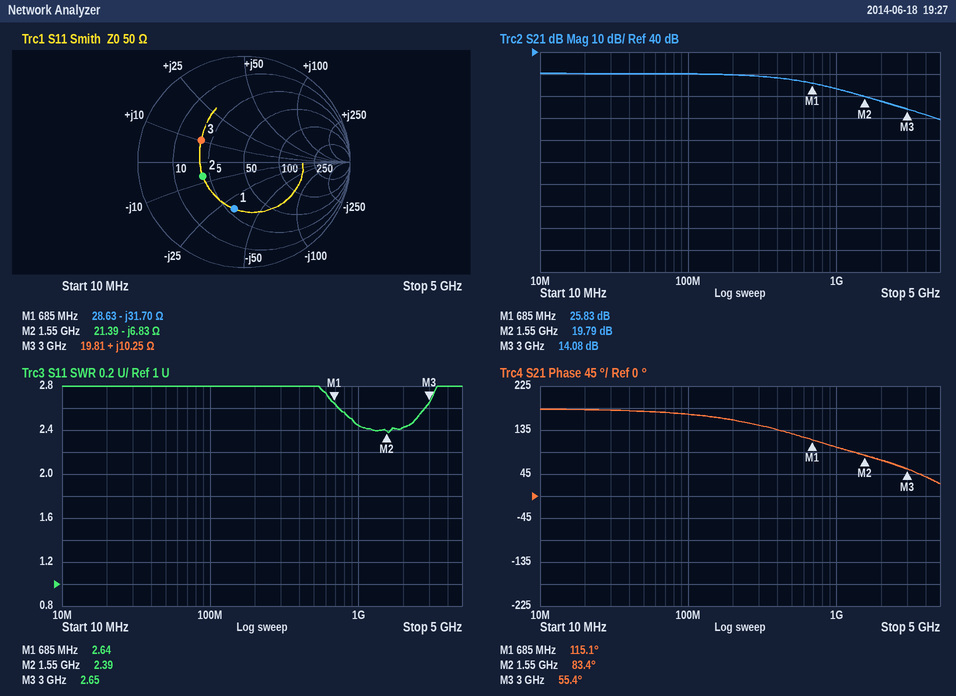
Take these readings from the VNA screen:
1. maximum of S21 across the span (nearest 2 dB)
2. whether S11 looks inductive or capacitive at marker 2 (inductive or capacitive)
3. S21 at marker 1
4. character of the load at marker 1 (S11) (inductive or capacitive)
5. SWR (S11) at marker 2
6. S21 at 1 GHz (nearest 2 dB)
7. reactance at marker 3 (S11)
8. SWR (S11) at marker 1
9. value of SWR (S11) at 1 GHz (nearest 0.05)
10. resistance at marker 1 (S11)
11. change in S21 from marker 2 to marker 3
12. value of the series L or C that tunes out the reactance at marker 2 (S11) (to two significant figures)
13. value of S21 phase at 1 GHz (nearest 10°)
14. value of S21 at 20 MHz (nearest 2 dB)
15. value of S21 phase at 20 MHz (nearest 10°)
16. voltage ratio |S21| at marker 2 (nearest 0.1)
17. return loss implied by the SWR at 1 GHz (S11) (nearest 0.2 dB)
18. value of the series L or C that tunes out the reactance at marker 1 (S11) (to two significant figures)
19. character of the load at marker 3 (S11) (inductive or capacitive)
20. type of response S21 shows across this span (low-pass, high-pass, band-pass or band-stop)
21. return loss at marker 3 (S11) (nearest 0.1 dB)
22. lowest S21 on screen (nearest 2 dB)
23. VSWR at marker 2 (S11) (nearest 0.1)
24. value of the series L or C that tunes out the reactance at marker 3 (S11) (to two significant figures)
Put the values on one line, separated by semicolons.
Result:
30 dB; capacitive; 25.83 dB; capacitive; 2.39; 24 dB; +10.25 Ω; 2.64; 2.45; 28.63 Ω; -5.71 dB; 700 pH; 100°; 30 dB; 180°; 9.8; 7.6 dB; 7.4 nH; inductive; low-pass; 6.9 dB; 10 dB; 2.4; 5.2 pF
